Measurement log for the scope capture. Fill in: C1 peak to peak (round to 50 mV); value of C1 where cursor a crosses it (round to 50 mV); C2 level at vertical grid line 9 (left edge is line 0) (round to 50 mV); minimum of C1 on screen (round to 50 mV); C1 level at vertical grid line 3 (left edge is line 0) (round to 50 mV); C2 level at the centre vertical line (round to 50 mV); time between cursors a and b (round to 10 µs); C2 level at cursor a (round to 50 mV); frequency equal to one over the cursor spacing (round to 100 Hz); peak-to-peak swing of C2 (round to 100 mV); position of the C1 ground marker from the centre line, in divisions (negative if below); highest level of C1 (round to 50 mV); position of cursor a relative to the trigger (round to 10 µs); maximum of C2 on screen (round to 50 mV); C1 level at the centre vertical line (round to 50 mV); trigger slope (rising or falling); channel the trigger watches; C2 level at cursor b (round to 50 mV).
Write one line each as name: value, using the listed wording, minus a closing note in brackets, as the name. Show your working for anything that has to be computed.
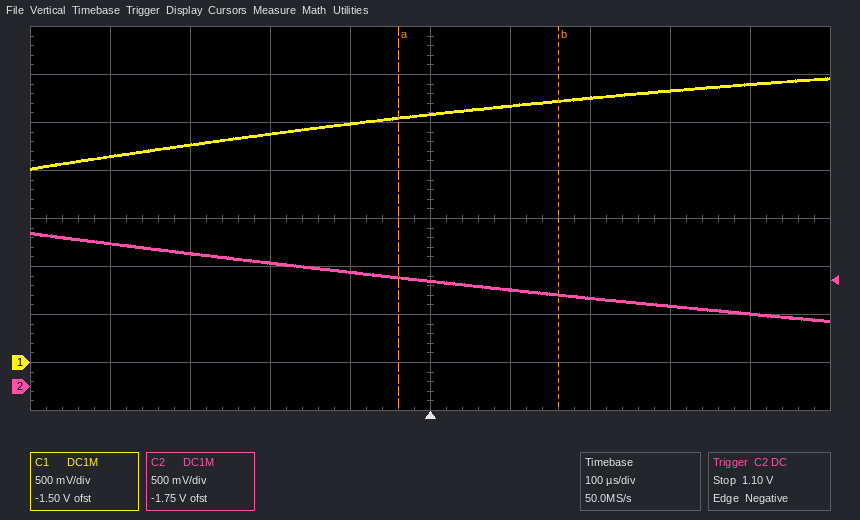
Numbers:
C1 peak to peak: 2.95 V − (2.00 V) = 950 mV
value of C1 where cursor a crosses it: 2.55 V
C2 level at vertical grid line 9 (left edge is line 0): 750 mV
minimum of C1 on screen: 2.00 V
C1 level at vertical grid line 3 (left edge is line 0): 2.40 V
C2 level at the centre vertical line: 1.10 V
time between cursors a and b: 200 µs
C2 level at cursor a: 1.15 V
frequency equal to one over the cursor spacing: 1 / 200 µs ≈ 5.0 kHz
peak-to-peak swing of C2: 900 mV
position of the C1 ground marker from the centre line, in divisions: -3.0 div
highest level of C1: 2.95 V
position of cursor a relative to the trigger: -40 µs
maximum of C2 on screen: 1.60 V
C1 level at the centre vertical line: 2.60 V
trigger slope: falling
channel the trigger watches: C2
C2 level at cursor b: 950 mV
